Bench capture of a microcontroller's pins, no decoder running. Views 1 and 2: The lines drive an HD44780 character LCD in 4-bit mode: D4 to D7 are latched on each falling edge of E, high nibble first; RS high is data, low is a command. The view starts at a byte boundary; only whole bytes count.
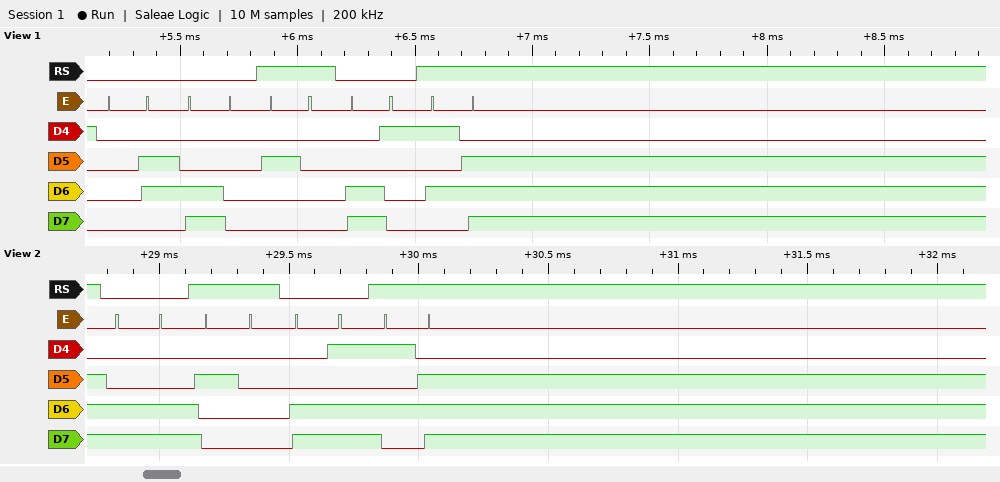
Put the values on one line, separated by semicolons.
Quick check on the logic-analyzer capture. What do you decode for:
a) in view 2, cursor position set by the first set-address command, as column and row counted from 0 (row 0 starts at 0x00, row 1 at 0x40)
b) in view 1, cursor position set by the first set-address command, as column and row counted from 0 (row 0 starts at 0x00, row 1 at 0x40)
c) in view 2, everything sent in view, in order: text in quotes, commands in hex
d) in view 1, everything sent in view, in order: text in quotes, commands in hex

column 12, row 1; column 0, row 1; 0xCC " " 0xCD "^"; 0x06 0xC0 " " 0xC1 "^"
